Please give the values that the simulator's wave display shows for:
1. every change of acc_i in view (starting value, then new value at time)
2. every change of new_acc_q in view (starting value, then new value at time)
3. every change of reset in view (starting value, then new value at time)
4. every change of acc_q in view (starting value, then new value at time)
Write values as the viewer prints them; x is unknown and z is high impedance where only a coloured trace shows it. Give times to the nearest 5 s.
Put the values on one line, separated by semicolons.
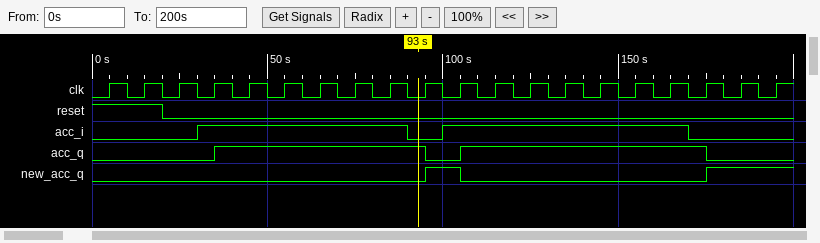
0, 1 at 30 s, 0 at 90 s, 1 at 100 s, 0 at 170 s; 0, 1 at 95 s, 0 at 105 s, 1 at 175 s; 1, 0 at 20 s; 0, 1 at 35 s, 0 at 95 s, 1 at 105 s, 0 at 175 s
